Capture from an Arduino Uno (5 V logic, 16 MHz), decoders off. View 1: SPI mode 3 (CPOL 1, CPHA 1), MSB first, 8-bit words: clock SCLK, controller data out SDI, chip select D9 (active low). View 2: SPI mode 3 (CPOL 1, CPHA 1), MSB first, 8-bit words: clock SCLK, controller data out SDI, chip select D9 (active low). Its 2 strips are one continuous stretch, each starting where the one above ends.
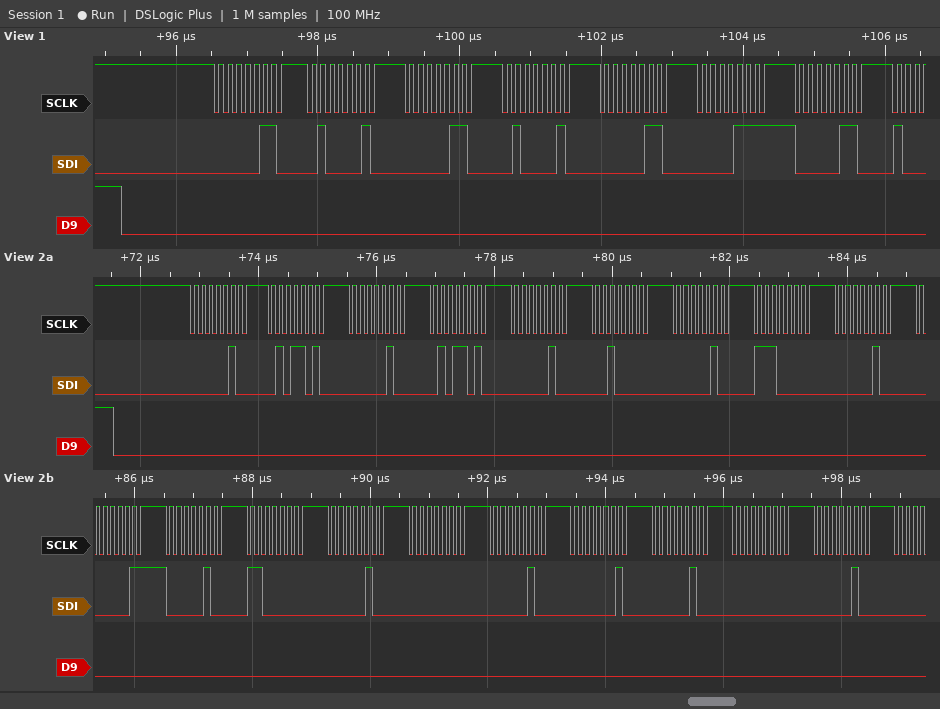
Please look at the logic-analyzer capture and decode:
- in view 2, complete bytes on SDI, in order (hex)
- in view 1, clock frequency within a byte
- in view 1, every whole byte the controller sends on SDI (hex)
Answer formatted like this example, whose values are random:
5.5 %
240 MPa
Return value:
04 5A 04 5A 04 20 04 E0 04 03 04 C0 04 00 04 02 04 00 04
8 MHz
0x06 0x42 0x06 0x42 0x06 0x0F 0x06
